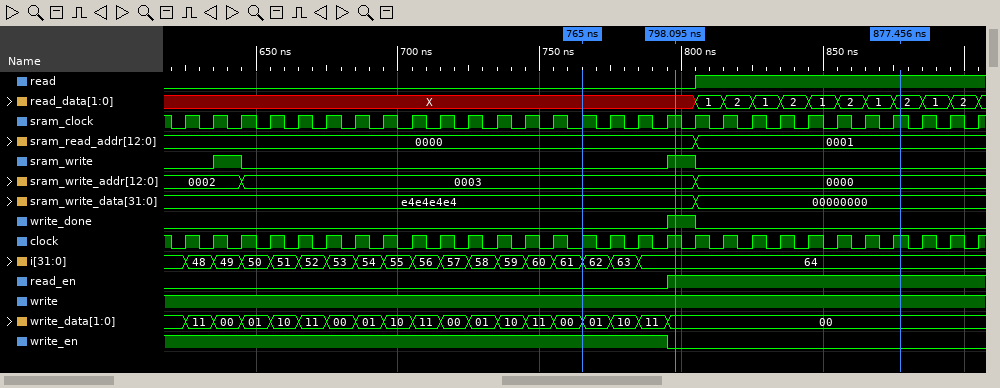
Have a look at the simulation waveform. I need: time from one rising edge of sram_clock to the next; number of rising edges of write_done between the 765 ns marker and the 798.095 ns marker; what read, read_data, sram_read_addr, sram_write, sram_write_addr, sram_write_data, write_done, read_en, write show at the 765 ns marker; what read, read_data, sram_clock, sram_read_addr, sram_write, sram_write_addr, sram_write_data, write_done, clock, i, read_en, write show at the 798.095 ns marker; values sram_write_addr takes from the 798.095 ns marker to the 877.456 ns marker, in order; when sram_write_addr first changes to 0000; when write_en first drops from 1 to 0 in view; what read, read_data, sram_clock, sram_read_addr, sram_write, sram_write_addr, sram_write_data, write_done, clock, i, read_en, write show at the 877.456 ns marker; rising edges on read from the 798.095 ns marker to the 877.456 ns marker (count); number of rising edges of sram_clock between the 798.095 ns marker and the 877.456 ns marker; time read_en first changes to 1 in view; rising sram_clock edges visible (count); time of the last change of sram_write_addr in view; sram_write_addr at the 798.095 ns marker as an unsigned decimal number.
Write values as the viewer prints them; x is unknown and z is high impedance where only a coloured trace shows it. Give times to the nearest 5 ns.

10 ns
1
read=0, read_data=X, sram_read_addr=0000, sram_write=0, sram_write_addr=0003, sram_write_data=e4e4e4e4, write_done=0, read_en=0, write=1
read=0, read_data=X, sram_clock=1, sram_read_addr=0000, sram_write=1, sram_write_addr=0003, sram_write_data=e4e4e4e4, write_done=1, clock=1, i=64, read_en=1, write=1
0003, 0000
805 ns
795 ns
read=1, read_data=2, sram_clock=1, sram_read_addr=0001, sram_write=0, sram_write_addr=0000, sram_write_data=00000000, write_done=0, clock=1, i=64, read_en=1, write=1
1
8
795 ns
29
805 ns
3
